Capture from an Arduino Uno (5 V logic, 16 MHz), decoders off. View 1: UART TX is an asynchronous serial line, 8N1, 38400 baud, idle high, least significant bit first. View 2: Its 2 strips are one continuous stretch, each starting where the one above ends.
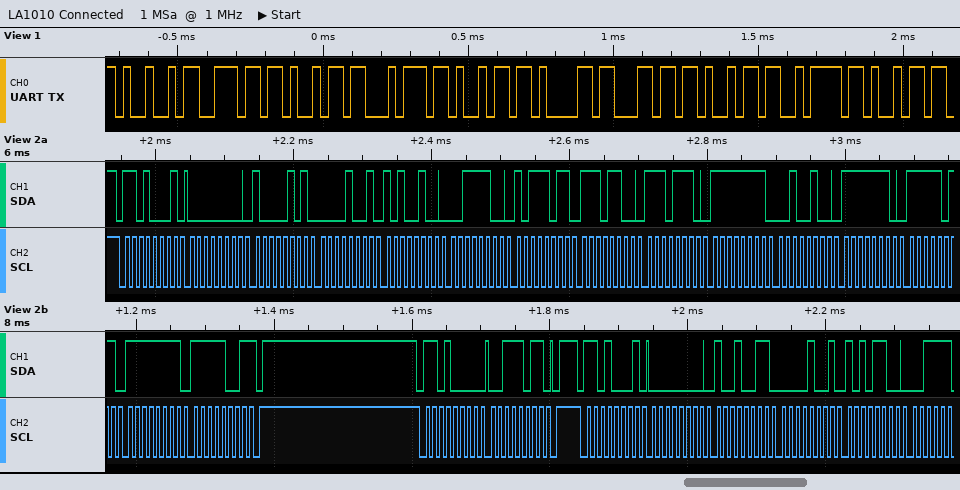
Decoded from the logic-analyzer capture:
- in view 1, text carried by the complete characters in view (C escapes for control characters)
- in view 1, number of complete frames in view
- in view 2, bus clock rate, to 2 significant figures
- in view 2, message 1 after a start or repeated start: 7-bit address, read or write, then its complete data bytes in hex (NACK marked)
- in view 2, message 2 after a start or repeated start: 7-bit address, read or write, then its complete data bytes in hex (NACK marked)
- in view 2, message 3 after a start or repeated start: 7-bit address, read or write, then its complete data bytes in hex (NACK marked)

"Initializi"
10
100 kHz
0x68 read: 00 85 09 A4 3C BB EC EE FF 24 FE FB FF F9 NACK
0x68 write: 3B
0x68 read: 00 93 09 AC
